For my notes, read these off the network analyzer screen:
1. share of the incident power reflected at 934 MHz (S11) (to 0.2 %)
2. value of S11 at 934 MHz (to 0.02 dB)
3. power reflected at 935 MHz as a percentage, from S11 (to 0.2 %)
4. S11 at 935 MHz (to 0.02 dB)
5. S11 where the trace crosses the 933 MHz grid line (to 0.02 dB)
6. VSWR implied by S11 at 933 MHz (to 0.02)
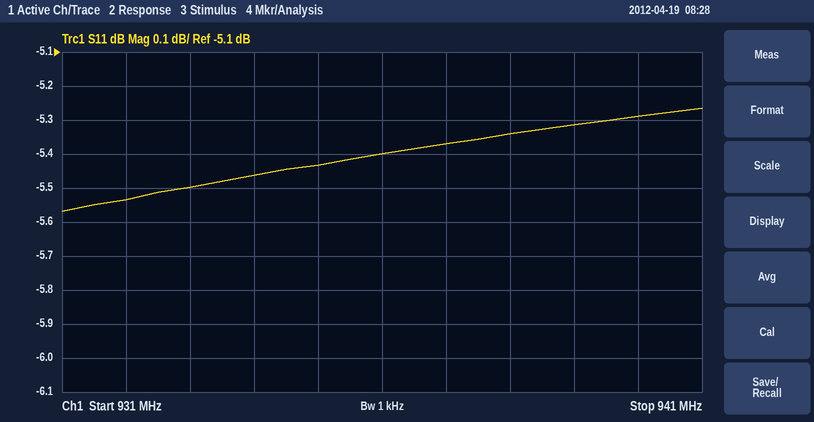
28.4 %
-5.46 dB
28.6 %
-5.44 dB
-5.50 dB
3.26
